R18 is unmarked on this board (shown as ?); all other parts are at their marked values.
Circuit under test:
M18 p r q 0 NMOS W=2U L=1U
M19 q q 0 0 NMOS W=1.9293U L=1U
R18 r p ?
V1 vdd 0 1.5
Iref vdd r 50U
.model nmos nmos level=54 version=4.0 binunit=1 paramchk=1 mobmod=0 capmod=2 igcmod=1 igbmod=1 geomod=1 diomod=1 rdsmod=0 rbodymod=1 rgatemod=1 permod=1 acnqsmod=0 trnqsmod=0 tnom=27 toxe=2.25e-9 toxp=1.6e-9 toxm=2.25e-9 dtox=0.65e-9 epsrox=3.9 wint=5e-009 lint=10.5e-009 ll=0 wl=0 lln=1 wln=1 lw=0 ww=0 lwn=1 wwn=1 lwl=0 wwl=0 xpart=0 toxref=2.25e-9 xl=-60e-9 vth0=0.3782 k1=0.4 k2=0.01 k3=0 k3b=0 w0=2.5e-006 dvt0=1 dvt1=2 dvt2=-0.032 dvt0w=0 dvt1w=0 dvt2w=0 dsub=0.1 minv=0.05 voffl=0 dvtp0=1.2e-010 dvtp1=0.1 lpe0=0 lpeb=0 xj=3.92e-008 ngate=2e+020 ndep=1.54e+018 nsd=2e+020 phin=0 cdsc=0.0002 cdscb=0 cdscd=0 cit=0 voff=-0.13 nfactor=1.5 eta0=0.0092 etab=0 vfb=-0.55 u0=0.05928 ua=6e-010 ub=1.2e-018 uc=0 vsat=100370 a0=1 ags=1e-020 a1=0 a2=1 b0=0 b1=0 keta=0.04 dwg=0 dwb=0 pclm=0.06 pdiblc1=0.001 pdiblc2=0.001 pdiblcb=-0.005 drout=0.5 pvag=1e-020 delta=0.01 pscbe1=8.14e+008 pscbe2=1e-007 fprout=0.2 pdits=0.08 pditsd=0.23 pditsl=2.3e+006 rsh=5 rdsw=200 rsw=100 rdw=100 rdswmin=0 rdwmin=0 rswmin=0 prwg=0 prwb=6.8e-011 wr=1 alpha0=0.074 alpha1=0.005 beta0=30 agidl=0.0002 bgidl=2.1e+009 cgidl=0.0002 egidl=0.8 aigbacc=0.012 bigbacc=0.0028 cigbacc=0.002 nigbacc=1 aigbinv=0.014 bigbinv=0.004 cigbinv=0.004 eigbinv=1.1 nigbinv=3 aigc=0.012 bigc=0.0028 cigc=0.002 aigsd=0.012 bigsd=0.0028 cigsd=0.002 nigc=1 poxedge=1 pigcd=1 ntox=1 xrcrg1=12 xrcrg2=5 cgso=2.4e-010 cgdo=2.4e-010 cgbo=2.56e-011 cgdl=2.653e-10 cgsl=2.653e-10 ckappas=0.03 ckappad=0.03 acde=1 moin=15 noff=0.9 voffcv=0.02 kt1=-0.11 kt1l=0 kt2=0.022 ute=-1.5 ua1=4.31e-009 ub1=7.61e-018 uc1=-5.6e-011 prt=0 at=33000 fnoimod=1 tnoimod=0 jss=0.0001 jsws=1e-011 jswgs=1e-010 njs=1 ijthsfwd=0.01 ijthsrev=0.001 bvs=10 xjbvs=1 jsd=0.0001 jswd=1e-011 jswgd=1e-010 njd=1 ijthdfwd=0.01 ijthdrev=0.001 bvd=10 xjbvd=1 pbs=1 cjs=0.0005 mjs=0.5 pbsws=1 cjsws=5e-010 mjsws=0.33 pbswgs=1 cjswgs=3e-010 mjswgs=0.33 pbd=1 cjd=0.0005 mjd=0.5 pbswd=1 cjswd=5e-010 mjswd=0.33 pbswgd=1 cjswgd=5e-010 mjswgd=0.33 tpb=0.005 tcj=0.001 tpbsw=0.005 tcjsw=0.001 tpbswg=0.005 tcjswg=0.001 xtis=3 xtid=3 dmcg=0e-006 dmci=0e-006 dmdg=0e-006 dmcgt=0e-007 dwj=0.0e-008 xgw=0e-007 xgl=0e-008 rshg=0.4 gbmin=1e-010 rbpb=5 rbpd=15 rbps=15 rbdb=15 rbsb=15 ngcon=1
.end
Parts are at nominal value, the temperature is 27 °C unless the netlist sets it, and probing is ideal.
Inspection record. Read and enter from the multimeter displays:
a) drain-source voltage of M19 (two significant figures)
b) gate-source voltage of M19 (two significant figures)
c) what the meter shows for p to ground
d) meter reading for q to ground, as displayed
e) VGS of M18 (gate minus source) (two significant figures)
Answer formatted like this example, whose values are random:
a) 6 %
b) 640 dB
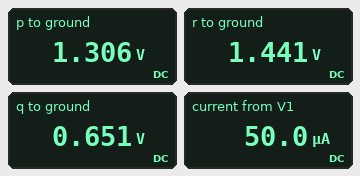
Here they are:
a) 650 mV
b) 650 mV
c) 1.306 V
d) 0.651 V
e) 790 mV
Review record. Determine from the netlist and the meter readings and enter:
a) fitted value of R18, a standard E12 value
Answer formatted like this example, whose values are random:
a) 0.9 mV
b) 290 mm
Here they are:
a) 2.7 kΩ
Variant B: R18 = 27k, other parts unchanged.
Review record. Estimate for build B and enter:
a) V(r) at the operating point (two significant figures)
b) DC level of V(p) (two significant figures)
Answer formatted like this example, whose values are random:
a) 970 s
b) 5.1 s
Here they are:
a) 2.1 V
b) 710 mV
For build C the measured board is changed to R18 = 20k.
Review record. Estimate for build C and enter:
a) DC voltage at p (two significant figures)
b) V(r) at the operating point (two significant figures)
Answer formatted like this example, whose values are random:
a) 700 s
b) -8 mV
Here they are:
a) 740 mV
b) 1.7 V
